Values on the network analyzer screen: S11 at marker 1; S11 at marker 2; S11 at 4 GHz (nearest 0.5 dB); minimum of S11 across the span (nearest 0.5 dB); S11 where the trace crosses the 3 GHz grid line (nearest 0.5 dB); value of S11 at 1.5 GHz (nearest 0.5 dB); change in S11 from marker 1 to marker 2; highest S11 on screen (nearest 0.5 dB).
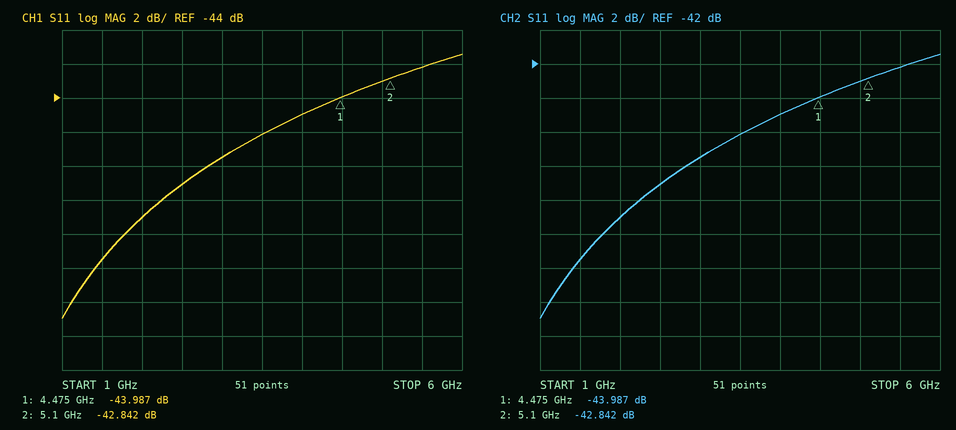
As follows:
-43.987 dB
-42.842 dB
-45.0 dB
-57.0 dB
-47.5 dB
-53.5 dB
1.145 dB
-41.5 dB
